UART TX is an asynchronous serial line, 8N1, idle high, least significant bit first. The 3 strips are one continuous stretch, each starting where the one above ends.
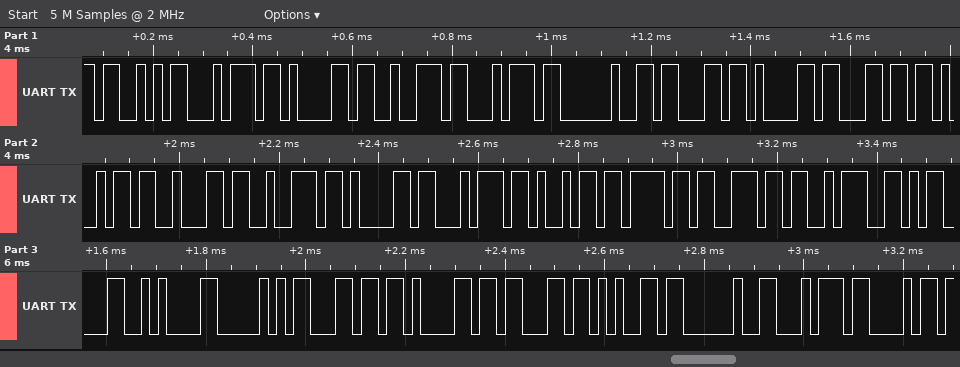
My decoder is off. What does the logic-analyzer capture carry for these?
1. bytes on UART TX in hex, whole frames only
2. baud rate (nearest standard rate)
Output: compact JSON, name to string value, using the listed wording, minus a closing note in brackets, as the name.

{"bytes on UART TX in hex, whole frames only": "53 74 61 72 74 20 63 61 6C 69 62 72 61 74 69 6F 6E 3A 0D 0A 50 6C 61 63 65 20 74 68", "baud rate": "57600 baud"}
